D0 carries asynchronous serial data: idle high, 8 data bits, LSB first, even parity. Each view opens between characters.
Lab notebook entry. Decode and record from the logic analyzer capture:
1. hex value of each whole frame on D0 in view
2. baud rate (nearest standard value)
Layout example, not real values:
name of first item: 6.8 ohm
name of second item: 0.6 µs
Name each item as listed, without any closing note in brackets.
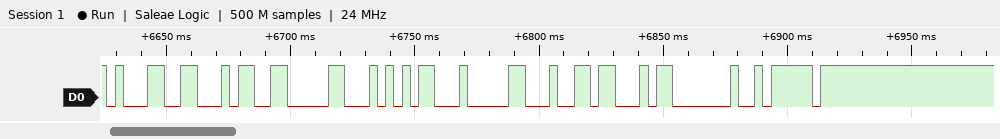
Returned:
hex value of each whole frame on D0 in view: 31, 34, 30, 35, 30, 36, 03, FA
baud rate: 300 baud
